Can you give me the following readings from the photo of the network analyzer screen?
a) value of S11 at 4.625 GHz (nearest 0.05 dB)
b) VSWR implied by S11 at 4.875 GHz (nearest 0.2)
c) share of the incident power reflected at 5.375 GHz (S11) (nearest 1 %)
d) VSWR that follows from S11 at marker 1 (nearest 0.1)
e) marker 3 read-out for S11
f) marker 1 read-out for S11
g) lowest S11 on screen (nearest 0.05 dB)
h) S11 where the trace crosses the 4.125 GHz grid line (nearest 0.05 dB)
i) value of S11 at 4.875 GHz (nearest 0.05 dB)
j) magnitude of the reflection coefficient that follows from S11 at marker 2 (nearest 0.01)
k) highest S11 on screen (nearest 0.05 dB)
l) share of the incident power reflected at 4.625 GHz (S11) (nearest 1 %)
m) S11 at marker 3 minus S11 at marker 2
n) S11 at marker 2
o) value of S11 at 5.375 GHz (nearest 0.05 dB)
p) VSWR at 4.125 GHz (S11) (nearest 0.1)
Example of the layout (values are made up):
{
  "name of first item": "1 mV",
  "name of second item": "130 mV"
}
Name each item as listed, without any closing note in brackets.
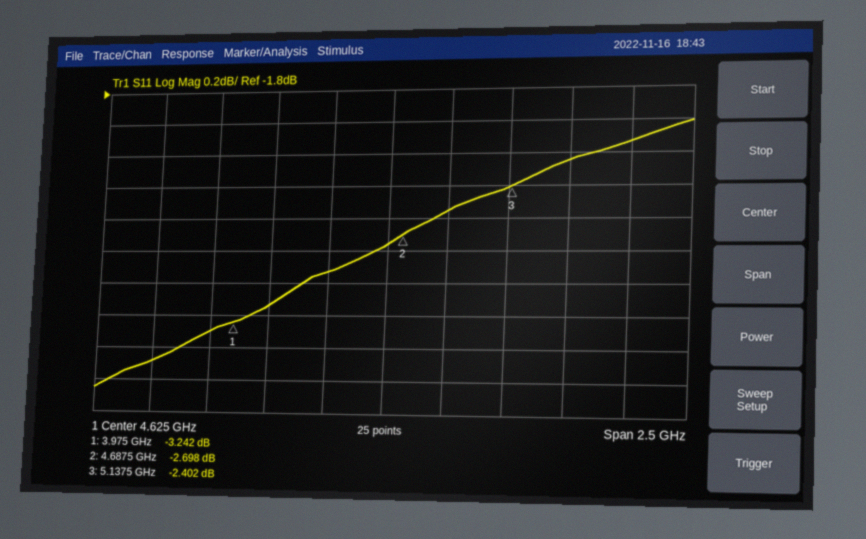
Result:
{
  "value of S11 at 4.625 GHz": "-2.75 dB",
  "VSWR implied by S11 at 4.875 GHz": "6.8",
  "share of the incident power reflected at 5.375 GHz (S11)": "60 %",
  "VSWR that follows from S11 at marker 1": "5.4",
  "marker 3 read-out for S11": "-2.402 dB",
  "marker 1 read-out for S11": "-3.242 dB",
  "lowest S11 on screen": "-3.65 dB",
  "S11 where the trace crosses the 4.125 GHz grid line": "-3.15 dB",
  "value of S11 at 4.875 GHz": "-2.55 dB",
  "magnitude of the reflection coefficient that follows from S11 at marker 2": "0.73",
  "highest S11 on screen": "-2.00 dB",
  "share of the incident power reflected at 4.625 GHz (S11)": "53 %",
  "S11 at marker 3 minus S11 at marker 2": "0.296 dB",
  "S11 at marker 2": "-2.698 dB",
  "value of S11 at 5.375 GHz": "-2.25 dB",
  "VSWR at 4.125 GHz (S11)": "5.6"
}
